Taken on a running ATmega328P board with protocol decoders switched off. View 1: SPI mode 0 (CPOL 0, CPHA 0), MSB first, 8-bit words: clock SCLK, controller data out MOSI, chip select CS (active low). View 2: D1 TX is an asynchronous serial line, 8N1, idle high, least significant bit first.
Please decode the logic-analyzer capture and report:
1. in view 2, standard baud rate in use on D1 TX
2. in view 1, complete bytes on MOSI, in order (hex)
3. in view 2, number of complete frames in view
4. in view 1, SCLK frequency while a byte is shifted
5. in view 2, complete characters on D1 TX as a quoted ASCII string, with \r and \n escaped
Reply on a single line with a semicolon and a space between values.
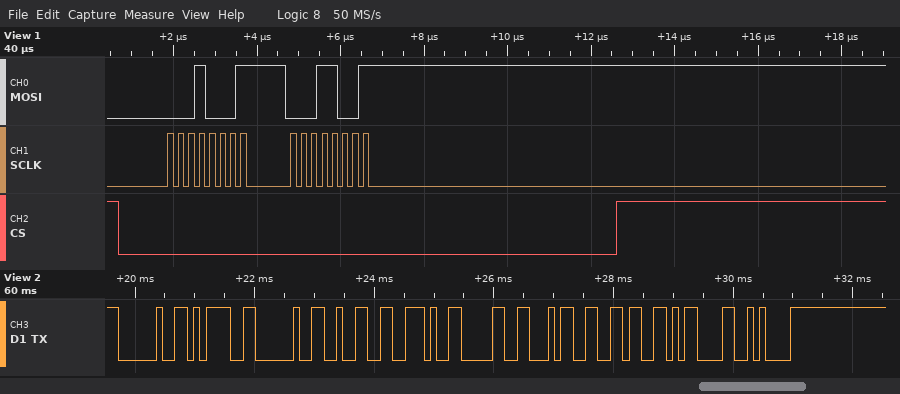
9600 baud; 11 19; 10; 4 MHz; " = 2.046\r\n"
